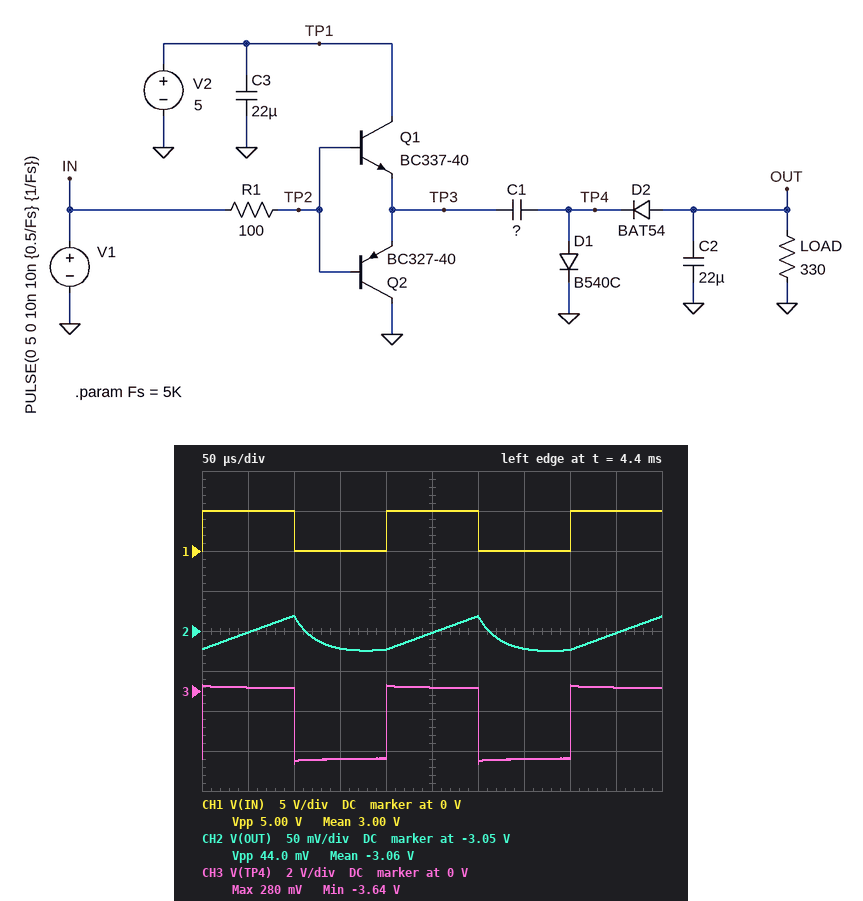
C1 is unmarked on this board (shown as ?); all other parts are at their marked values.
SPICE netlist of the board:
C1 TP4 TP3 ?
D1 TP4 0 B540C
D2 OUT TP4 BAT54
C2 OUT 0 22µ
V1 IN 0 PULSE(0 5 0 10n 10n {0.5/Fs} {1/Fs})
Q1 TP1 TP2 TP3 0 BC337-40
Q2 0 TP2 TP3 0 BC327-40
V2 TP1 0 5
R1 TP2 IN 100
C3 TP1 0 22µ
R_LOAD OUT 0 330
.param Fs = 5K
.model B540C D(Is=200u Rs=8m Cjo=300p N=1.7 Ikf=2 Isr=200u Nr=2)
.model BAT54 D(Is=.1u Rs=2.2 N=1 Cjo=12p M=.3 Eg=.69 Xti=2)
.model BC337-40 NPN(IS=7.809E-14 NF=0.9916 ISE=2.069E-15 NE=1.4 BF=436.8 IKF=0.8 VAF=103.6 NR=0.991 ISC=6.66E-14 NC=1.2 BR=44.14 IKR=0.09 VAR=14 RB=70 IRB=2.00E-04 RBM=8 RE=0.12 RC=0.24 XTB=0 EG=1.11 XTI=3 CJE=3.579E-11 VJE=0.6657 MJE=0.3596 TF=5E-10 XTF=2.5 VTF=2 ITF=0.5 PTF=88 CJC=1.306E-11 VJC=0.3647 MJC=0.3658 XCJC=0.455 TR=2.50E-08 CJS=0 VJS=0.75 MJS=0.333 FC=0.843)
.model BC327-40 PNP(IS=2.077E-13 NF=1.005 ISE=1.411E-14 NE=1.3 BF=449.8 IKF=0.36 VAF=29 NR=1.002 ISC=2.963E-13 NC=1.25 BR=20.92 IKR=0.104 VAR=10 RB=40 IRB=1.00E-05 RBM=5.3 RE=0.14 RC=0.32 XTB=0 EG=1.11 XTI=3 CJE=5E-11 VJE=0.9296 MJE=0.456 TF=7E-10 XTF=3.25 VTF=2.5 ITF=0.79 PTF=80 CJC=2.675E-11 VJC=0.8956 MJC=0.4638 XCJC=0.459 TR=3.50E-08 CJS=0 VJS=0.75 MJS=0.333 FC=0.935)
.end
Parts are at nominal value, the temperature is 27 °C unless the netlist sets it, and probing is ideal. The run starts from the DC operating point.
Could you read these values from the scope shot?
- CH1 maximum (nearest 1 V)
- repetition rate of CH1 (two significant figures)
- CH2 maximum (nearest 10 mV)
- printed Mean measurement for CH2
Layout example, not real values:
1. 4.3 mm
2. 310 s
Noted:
1. 5 V
2. 5.0 kHz
3. -3.03 V
4. -3.06 V
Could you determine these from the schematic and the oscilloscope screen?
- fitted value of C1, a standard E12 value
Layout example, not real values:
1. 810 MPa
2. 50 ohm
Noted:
1. 10 µF
